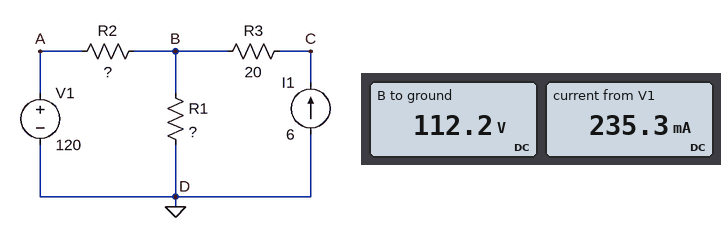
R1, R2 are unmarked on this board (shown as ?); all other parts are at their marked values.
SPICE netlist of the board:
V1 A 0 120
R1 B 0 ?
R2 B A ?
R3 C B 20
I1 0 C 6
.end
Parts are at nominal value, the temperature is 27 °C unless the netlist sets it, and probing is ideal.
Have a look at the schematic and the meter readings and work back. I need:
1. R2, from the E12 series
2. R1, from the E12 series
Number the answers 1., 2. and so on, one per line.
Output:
1. 33 Ω
2. 18 Ω
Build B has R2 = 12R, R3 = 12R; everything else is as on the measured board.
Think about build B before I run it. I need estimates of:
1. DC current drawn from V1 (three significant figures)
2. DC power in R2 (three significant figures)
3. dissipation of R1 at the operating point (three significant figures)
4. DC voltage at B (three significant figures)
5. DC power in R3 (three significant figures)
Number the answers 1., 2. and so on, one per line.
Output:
1. 400 mA
2. 1.92 W
3. 737 W
4. 115 V
5. 432 W
